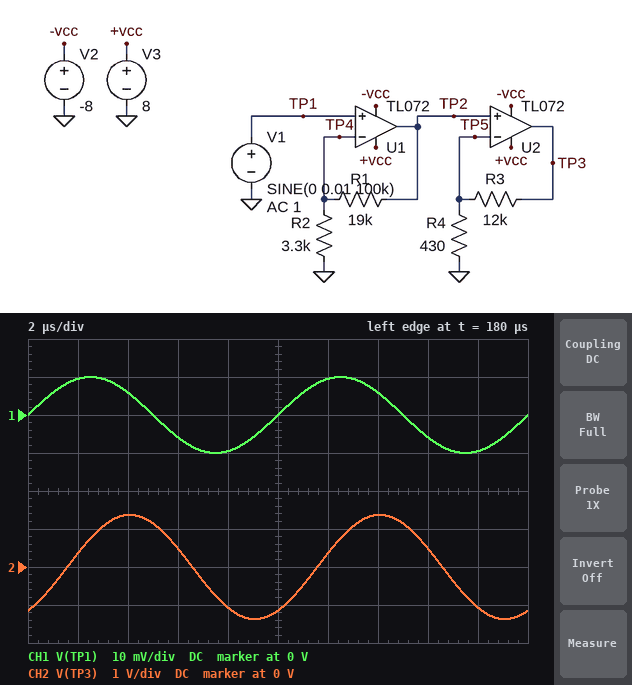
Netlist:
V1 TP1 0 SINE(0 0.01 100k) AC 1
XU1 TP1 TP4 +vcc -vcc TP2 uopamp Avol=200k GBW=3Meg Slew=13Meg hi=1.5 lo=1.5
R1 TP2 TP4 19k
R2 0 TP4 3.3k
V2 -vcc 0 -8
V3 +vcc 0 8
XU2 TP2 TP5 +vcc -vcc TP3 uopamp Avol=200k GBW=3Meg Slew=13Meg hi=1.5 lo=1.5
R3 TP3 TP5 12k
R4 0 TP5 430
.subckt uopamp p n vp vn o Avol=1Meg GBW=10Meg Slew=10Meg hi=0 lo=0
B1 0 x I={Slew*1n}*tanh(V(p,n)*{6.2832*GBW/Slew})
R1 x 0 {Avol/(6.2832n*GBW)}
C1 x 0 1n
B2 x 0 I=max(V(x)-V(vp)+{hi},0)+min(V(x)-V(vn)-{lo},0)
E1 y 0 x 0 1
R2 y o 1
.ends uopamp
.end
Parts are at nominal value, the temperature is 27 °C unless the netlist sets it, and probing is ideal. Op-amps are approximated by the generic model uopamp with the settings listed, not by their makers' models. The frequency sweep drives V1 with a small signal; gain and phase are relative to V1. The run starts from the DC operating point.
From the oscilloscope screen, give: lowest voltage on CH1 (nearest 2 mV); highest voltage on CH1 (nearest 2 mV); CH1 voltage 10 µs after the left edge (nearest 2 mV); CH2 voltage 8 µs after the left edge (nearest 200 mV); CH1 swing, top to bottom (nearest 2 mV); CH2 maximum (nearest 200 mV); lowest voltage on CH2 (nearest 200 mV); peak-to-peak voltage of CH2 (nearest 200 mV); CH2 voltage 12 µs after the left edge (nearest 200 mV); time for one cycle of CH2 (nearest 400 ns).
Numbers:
-10 mV
10 mV
0 V
-1.0 V
20 mV
1.4 V
-1.4 V
2.8 V
400 mV
10.0 µs
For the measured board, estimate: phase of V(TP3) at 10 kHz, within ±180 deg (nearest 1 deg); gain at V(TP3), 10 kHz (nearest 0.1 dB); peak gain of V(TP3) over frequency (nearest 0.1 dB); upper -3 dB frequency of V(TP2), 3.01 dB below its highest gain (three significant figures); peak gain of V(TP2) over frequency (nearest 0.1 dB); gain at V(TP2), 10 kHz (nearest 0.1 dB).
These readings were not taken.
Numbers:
-7 deg
45.8 dB
45.8 dB
444 kHz
16.6 dB
16.6 dB
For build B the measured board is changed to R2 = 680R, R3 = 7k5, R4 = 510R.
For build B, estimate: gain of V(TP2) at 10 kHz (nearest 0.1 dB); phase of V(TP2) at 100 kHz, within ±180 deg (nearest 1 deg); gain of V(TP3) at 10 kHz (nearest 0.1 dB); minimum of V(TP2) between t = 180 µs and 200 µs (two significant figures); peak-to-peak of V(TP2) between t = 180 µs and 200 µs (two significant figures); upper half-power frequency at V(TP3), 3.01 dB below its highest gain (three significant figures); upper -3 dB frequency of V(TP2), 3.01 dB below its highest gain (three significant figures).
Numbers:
29.2 dB
-44 deg
53.1 dB
-210 mV
420 mV
84.9 kHz
104 kHz
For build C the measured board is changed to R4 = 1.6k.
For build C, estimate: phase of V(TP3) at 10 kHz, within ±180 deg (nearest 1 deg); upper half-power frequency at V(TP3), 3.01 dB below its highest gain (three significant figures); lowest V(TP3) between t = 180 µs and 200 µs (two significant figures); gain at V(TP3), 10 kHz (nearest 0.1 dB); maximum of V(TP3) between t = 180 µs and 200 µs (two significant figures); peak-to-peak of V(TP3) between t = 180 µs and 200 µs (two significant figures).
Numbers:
-3 deg
252 kHz
-540 mV
35.2 dB
540 mV
1.1 V
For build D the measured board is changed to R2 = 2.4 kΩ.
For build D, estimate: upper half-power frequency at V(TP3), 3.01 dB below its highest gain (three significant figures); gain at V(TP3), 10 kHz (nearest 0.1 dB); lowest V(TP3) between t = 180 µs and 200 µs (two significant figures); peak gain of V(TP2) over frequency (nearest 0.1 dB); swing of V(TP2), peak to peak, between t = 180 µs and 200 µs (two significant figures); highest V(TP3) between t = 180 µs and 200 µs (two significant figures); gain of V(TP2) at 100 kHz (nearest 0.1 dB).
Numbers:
95.7 kHz
48.2 dB
-1.8 V
19.0 dB
170 mV
1.8 V
18.6 dB
